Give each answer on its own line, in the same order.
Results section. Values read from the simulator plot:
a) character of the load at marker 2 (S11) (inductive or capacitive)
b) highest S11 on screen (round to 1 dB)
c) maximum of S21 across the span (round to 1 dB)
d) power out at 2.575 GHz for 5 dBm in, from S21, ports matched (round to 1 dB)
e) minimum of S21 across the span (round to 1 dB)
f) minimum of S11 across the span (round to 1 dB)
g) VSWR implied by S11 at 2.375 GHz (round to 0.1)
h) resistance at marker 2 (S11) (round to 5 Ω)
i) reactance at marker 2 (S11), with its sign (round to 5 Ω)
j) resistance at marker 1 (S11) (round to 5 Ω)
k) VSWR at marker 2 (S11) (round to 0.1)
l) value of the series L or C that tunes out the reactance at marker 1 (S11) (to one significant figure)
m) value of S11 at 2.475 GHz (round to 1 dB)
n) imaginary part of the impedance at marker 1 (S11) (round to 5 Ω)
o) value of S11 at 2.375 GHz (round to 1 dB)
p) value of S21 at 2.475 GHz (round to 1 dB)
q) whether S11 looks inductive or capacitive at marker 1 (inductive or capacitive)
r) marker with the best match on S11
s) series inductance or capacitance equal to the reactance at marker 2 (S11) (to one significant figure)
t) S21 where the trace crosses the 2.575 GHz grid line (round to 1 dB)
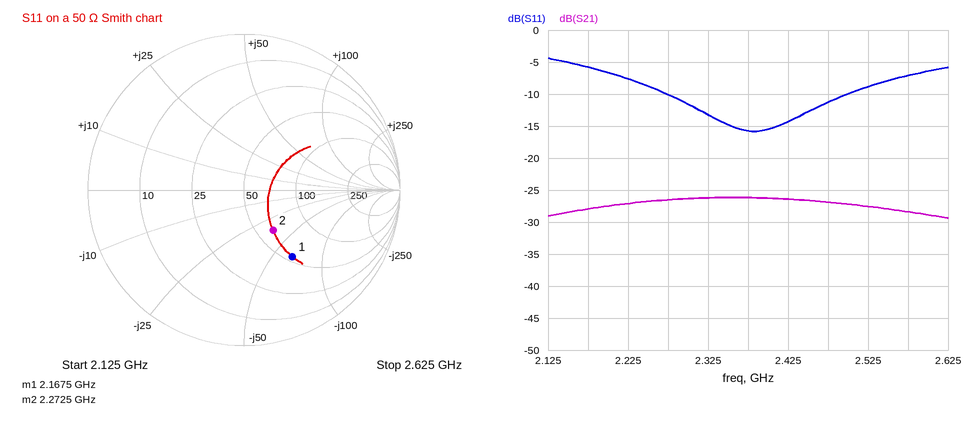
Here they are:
capacitive
-4 dB
-26 dB
-23 dBm
-29 dB
-16 dB
1.4
60 Ω
-35 Ω
55 Ω
1.9
5 nH
-11 dB
-65 Ω
-16 dB
-27 dB
capacitive
marker 2
2 pF
-28 dB
